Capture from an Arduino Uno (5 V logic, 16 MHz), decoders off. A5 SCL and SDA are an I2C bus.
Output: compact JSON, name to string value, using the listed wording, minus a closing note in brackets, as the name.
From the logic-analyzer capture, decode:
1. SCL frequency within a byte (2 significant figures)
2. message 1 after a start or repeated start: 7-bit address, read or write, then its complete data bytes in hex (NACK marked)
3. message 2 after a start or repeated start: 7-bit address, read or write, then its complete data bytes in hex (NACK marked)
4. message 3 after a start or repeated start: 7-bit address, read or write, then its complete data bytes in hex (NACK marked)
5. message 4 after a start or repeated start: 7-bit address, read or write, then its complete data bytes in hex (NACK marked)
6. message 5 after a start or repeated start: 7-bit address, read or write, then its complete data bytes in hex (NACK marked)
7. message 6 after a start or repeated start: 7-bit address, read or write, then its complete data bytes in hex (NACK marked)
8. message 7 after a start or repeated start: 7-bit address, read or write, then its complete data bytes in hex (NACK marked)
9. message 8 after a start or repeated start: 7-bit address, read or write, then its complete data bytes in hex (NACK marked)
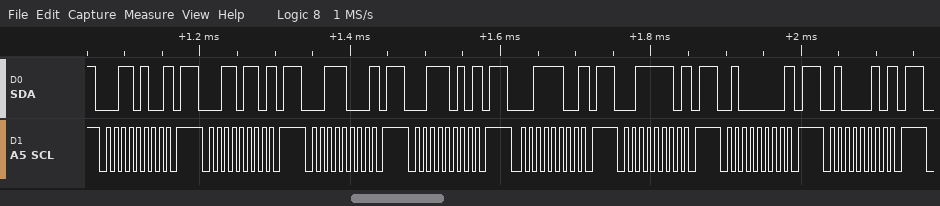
{"SCL frequency within a byte": "100 kHz", "message 1 after a start or repeated start: 7-bit address, read or write, then its complete data bytes in hex": "0x1A write NACK", "message 2 after a start or repeated start: 7-bit address, read or write, then its complete data bytes in hex": "0x1B write NACK", "message 3 after a start or repeated start: 7-bit address, read or write, then its complete data bytes in hex": "0x1C write NACK", "message 4 after a start or repeated start: 7-bit address, read or write, then its complete data bytes in hex": "0x1D write NACK", "message 5 after a start or repeated start: 7-bit address, read or write, then its complete data bytes in hex": "0x1E write NACK", "message 6 after a start or repeated start: 7-bit address, read or write, then its complete data bytes in hex": "0x1F write NACK", "message 7 after a start or repeated start: 7-bit address, read or write, then its complete data bytes in hex": "0x20 write NACK", "message 8 after a start or repeated start: 7-bit address, read or write, then its complete data bytes in hex": "0x21 write NACK"}
